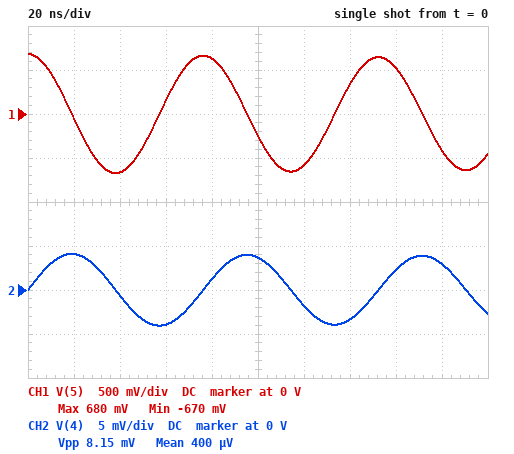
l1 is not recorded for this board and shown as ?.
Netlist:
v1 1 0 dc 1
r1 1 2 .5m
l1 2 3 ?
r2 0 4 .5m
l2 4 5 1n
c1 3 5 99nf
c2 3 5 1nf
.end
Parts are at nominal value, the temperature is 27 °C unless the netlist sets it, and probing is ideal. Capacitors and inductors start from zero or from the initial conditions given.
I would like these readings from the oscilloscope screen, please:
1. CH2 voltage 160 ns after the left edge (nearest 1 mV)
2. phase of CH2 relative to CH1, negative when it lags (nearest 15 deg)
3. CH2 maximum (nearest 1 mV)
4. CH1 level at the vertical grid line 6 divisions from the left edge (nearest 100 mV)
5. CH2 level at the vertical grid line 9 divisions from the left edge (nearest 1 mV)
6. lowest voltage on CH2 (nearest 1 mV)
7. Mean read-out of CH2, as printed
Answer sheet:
2 mV
-90 deg
4 mV
-600 mV
3 mV
-4 mV
400 µV
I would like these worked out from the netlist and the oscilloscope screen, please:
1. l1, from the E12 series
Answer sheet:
470 pH
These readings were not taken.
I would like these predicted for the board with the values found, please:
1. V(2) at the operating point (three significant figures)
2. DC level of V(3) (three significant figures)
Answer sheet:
1.00 V
1.00 V
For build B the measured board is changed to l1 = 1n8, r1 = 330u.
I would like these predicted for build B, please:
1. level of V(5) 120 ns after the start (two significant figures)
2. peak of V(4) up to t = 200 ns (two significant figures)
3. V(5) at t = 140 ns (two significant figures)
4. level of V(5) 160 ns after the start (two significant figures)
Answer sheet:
220 mV
3.0 mV
-170 mV
-350 mV
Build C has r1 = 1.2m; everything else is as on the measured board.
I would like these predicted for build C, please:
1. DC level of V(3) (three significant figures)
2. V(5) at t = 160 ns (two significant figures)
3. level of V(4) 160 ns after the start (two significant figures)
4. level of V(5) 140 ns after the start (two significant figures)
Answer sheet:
1.00 V
500 mV
2.2 mV
330 mV
